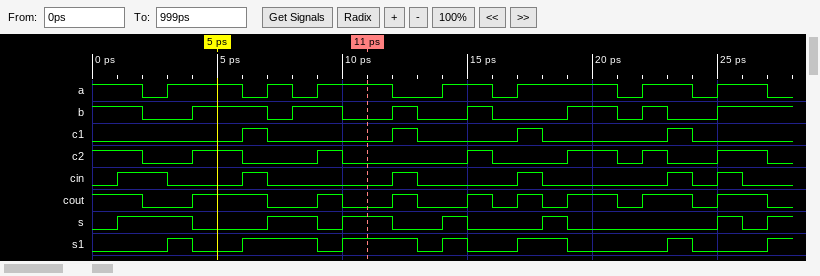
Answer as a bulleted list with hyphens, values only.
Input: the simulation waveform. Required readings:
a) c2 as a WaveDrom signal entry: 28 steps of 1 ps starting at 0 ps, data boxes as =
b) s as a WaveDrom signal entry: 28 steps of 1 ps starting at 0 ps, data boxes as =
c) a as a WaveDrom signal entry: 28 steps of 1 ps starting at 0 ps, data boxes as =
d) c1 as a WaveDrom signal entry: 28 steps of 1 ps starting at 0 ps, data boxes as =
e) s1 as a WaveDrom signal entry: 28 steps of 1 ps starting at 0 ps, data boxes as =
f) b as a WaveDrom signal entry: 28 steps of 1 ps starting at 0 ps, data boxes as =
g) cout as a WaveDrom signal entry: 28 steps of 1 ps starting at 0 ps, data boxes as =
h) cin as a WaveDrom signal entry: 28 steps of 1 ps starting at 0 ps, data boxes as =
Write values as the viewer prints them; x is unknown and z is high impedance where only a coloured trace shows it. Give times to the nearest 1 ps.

- {name: 'c2', wave: '1.0.1.0..10....10..1.010.1.0'}
- {name: 's', wave: '01..0..1.01.0.10..10.....101'}
- {name: 'a', wave: '1.01..0101..0.1.01...01.01.0'}
- {name: 'c1', wave: '0.....10....10...10....10...'}
- {name: 's1', wave: '0..10.1..01..010.1.0...10..1'}
- {name: 'b', wave: '1.0.1..01.0.10.10..1.010.1..'}
- {name: 'cout', wave: '1.0.1..0.10.10.10101.01.01.0'}
- {name: 'cin', wave: '01.0..10....10...10....1010.'}
